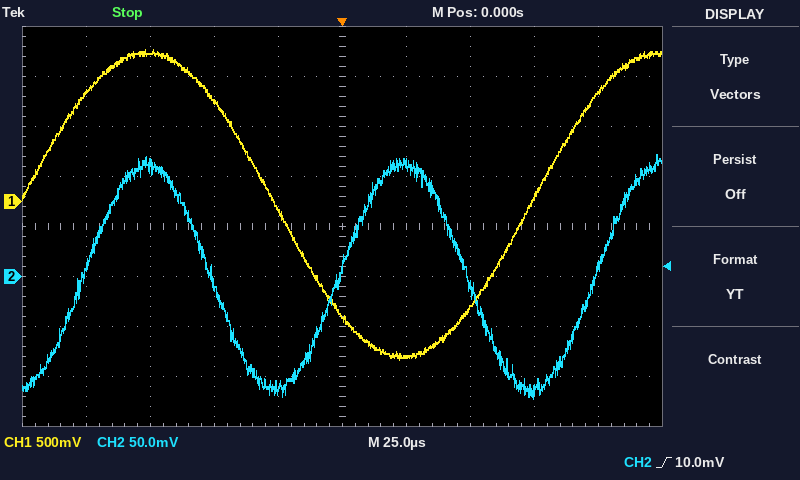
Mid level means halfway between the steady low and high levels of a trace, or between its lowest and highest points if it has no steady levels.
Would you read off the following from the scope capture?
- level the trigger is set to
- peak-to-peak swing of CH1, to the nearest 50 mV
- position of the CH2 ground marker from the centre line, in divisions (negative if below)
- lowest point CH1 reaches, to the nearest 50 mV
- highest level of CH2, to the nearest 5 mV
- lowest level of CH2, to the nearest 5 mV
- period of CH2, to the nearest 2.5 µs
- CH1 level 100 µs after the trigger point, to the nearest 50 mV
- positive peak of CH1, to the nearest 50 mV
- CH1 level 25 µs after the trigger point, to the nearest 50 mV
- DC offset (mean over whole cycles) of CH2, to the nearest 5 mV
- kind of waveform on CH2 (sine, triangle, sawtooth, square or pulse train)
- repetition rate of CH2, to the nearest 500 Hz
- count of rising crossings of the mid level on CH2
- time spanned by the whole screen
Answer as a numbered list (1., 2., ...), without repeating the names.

1. 10.0 mV
2. 3.10 V
3. -1.0 div
4. -1.60 V
5. 120 mV
6. -120 mV
7. 100.0 µs
8. 1.10 V
9. 1.50 V
10. -1.55 V
11. 0 mV
12. sine
13. 10.0 kHz
14. 3
15. 250 µs
